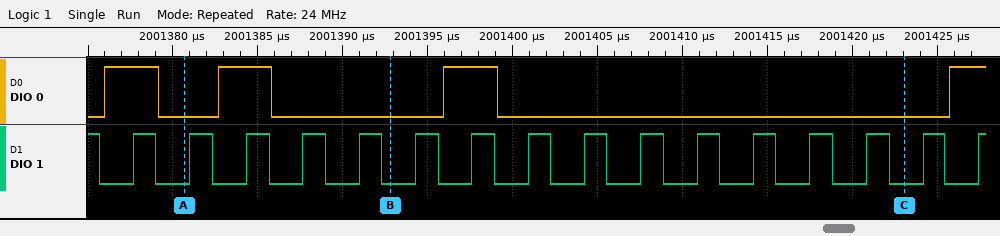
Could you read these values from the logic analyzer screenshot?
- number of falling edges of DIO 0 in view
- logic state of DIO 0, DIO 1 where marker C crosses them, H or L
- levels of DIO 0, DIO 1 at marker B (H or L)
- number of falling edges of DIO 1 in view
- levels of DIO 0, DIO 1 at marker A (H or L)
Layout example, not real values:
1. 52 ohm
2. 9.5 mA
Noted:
1. 3
2. DIO 0=L, DIO 1=L
3. DIO 0=L, DIO 1=L
4. 16
5. DIO 0=L, DIO 1=L
